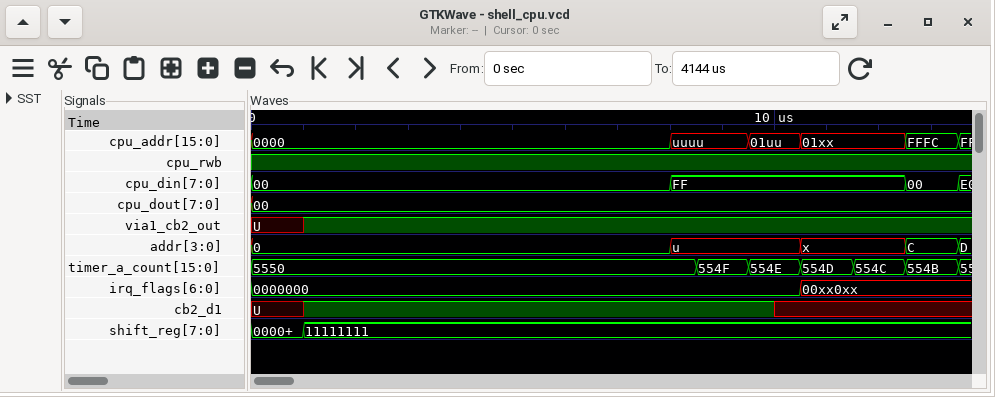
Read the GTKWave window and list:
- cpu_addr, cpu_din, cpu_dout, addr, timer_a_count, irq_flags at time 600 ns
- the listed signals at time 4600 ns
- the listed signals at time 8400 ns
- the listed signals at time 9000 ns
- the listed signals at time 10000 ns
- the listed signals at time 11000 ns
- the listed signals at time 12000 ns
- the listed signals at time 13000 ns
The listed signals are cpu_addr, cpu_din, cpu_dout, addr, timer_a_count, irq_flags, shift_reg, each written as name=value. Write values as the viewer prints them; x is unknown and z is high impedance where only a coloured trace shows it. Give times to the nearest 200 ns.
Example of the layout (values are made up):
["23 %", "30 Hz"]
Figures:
["cpu_addr=0000, cpu_din=00, cpu_dout=00, addr=0, timer_a_count=5550, irq_flags=0000000", "cpu_addr=0000, cpu_din=00, cpu_dout=00, addr=0, timer_a_count=5550, irq_flags=0000000, shift_reg=11111111", "cpu_addr=uuuu, cpu_din=FF, cpu_dout=00, addr=u, timer_a_count=5550, irq_flags=0000000, shift_reg=11111111", "cpu_addr=uuuu, cpu_din=FF, cpu_dout=00, addr=u, timer_a_count=554F, irq_flags=0000000, shift_reg=11111111", "cpu_addr=01uu, cpu_din=FF, cpu_dout=00, addr=u, timer_a_count=554E, irq_flags=0000000, shift_reg=11111111", "cpu_addr=01xx, cpu_din=FF, cpu_dout=00, addr=x, timer_a_count=554D, irq_flags=00xx0xx, shift_reg=11111111", "cpu_addr=01xx, cpu_din=FF, cpu_dout=00, addr=x, timer_a_count=554C, irq_flags=00xx0xx, shift_reg=11111111", "cpu_addr=FFFC, cpu_din=00, cpu_dout=00, addr=C, timer_a_count=554B, irq_flags=00xx0xx, shift_reg=11111111"]
